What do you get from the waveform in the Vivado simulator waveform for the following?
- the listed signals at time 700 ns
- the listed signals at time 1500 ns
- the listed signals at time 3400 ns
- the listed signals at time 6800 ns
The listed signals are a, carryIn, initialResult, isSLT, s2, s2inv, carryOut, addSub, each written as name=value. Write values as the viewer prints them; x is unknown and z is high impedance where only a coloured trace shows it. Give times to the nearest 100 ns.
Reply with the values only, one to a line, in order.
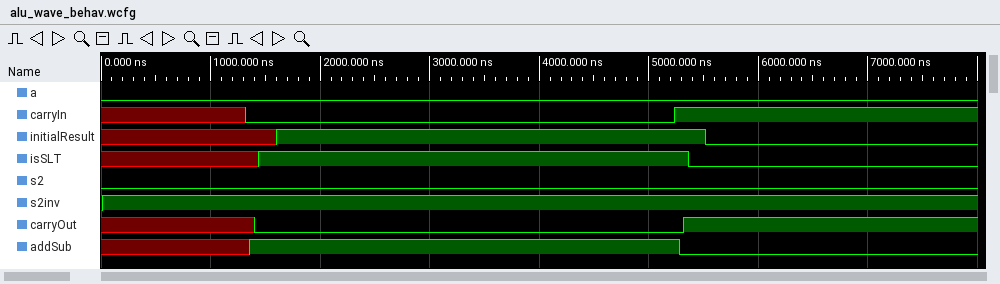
a=0, carryIn=x, initialResult=x, isSLT=x, s2=0, s2inv=1, carryOut=x, addSub=x
a=0, carryIn=0, initialResult=x, isSLT=1, s2=0, s2inv=1, carryOut=0, addSub=1
a=0, carryIn=0, initialResult=1, isSLT=1, s2=0, s2inv=1, carryOut=0, addSub=1
a=0, carryIn=1, initialResult=0, isSLT=0, s2=0, s2inv=1, carryOut=1, addSub=0
